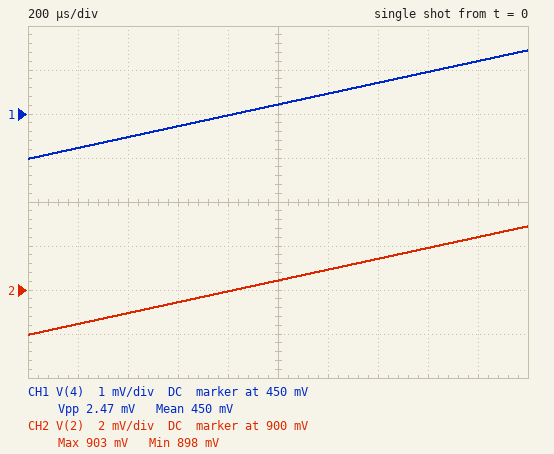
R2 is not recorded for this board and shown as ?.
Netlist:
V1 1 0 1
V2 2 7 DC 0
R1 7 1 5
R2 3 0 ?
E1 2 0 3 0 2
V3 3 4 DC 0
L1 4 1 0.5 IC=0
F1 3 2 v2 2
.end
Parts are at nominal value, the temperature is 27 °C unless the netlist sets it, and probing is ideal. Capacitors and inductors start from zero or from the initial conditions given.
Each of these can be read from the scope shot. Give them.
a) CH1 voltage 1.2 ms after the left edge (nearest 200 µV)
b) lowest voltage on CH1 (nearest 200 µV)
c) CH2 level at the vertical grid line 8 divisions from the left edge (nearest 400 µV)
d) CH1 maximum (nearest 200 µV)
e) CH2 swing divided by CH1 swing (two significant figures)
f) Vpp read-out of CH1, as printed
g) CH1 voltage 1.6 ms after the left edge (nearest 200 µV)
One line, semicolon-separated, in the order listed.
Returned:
450.4 mV; 449.0 mV; 902.0 mV; 451.4 mV; 2.0; 2.47 mV; 451.0 mV
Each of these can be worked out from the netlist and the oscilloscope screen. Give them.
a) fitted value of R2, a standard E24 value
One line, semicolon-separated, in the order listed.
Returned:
11 Ω
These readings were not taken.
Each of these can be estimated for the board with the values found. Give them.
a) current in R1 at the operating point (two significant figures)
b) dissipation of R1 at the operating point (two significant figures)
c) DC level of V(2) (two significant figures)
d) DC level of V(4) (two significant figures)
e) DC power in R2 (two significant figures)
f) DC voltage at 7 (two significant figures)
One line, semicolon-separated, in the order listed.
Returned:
200 mA; 200 mW; 2.0 V; 1.0 V; 91 mW; 2.0 V
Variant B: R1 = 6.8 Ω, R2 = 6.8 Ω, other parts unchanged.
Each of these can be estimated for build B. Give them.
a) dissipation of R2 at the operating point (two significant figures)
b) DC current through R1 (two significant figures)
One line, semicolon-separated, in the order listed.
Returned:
150 mW; 150 mA
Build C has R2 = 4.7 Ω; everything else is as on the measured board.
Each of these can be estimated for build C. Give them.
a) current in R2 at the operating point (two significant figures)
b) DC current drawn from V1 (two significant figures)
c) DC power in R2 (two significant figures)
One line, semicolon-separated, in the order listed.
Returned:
210 mA; 410 mA; 210 mW
